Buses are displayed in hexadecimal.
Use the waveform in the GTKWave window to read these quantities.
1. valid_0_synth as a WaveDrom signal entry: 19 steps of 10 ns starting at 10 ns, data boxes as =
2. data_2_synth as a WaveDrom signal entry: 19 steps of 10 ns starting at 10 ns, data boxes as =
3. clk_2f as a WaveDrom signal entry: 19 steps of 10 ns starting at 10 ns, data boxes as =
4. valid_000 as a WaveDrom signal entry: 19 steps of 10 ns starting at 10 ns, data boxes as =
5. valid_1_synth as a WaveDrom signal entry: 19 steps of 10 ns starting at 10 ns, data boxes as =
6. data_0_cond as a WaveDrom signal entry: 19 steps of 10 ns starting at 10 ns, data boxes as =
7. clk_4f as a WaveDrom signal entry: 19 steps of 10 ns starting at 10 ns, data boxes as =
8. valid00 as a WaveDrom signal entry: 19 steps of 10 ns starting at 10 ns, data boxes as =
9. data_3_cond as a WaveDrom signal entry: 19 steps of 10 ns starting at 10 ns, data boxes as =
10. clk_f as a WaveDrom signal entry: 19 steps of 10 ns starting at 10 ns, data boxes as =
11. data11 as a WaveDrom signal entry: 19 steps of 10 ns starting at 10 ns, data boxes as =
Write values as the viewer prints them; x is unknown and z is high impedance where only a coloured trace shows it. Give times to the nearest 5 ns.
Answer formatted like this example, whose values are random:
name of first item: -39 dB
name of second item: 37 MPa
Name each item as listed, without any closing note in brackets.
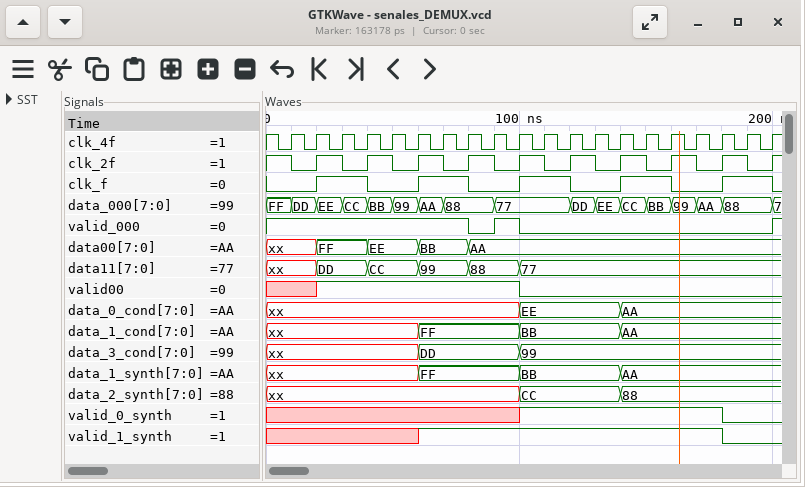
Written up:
valid_0_synth as a WaveDrom signal entry: 19 steps of 10 ns starting at 10 ns, data boxes as =: {name: 'valid_0_synth', wave: 'x........1.......0.'}
data_2_synth as a WaveDrom signal entry: 19 steps of 10 ns starting at 10 ns, data boxes as =: {name: 'data_2_synth', wave: 'x........=...=.....', data: 'CC 88'}
clk_2f as a WaveDrom signal entry: 19 steps of 10 ns starting at 10 ns, data boxes as =: {name: 'clk_2f', wave: '0101010101010101010'}
valid_000 as a WaveDrom signal entry: 19 steps of 10 ns starting at 10 ns, data boxes as =: {name: 'valid_000', wave: '1......010.........'}
valid_1_synth as a WaveDrom signal entry: 19 steps of 10 ns starting at 10 ns, data boxes as =: {name: 'valid_1_synth', wave: 'x....1...........0.'}
data_0_cond as a WaveDrom signal entry: 19 steps of 10 ns starting at 10 ns, data boxes as =: {name: 'data_0_cond', wave: 'x........=...=.....', data: 'EE AA'}
clk_4f as a WaveDrom signal entry: 19 steps of 10 ns starting at 10 ns, data boxes as =: {name: 'clk_4f', wave: 'p..................'}
valid00 as a WaveDrom signal entry: 19 steps of 10 ns starting at 10 ns, data boxes as =: {name: 'valid00', wave: 'x1.......0.........'}
data_3_cond as a WaveDrom signal entry: 19 steps of 10 ns starting at 10 ns, data boxes as =: {name: 'data_3_cond', wave: 'x....=...=.........', data: 'DD 99'}
clk_f as a WaveDrom signal entry: 19 steps of 10 ns starting at 10 ns, data boxes as =: {name: 'clk_f', wave: '01.0.1.0.1.0.1.0.1.'}
data11 as a WaveDrom signal entry: 19 steps of 10 ns starting at 10 ns, data boxes as =: {name: 'data11', wave: 'x=.=.=.=.=.........', data: 'DD CC 99 88 77'}
